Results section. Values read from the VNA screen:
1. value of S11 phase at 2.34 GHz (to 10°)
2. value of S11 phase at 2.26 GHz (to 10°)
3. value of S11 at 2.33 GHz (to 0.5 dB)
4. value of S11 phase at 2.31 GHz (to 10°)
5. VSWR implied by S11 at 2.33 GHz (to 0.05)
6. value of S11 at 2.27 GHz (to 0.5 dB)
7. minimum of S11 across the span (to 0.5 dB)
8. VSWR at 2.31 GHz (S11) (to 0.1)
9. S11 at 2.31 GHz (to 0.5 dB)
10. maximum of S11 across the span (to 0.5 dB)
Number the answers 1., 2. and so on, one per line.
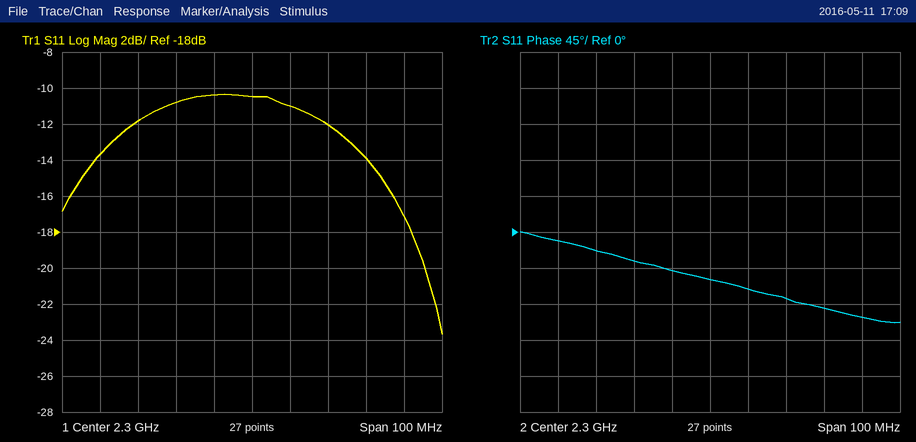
1. -110°
2. -10°
3. -14.0 dB
4. -70°
5. 1.50
6. -12.0 dB
7. -23.5 dB
8. 1.8
9. -11.0 dB
10. -10.5 dB
